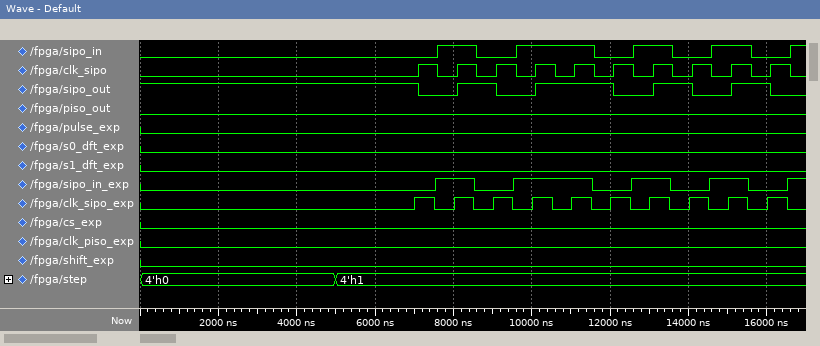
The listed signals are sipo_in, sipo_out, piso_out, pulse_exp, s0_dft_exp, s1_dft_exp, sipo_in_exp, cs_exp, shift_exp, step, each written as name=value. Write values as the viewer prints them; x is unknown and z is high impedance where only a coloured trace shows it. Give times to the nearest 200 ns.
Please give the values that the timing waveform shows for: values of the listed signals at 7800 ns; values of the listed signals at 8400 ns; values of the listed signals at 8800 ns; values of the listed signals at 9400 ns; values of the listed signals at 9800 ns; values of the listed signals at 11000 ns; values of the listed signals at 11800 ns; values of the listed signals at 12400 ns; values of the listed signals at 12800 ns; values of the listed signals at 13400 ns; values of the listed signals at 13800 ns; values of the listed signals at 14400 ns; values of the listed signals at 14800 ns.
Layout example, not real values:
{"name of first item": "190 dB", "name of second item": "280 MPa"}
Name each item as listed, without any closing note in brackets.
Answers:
{"values of the listed signals at 7800 ns": "sipo_in=1, sipo_out=0, piso_out=0, pulse_exp=0, s0_dft_exp=0, s1_dft_exp=0, sipo_in_exp=1, cs_exp=0, shift_exp=0, step=4'h1", "values of the listed signals at 8400 ns": "sipo_in=1, sipo_out=1, piso_out=0, pulse_exp=0, s0_dft_exp=0, s1_dft_exp=0, sipo_in_exp=1, cs_exp=0, shift_exp=0, step=4'h1", "values of the listed signals at 8800 ns": "sipo_in=0, sipo_out=1, piso_out=0, pulse_exp=0, s0_dft_exp=0, s1_dft_exp=0, sipo_in_exp=0, cs_exp=0, shift_exp=0, step=4'h1", "values of the listed signals at 9400 ns": "sipo_in=0, sipo_out=0, piso_out=0, pulse_exp=0, s0_dft_exp=0, s1_dft_exp=0, sipo_in_exp=0, cs_exp=0, shift_exp=0, step=4'h1", "values of the listed signals at 9800 ns": "sipo_in=1, sipo_out=0, piso_out=0, pulse_exp=0, s0_dft_exp=0, s1_dft_exp=0, sipo_in_exp=1, cs_exp=0, shift_exp=0, step=4'h1", "values of the listed signals at 11000 ns": "sipo_in=1, sipo_out=1, piso_out=0, pulse_exp=0, s0_dft_exp=0, s1_dft_exp=0, sipo_in_exp=1, cs_exp=0, shift_exp=0, step=4'h1", "values of the listed signals at 11800 ns": "sipo_in=0, sipo_out=1, piso_out=0, pulse_exp=0, s0_dft_exp=0, s1_dft_exp=0, sipo_in_exp=0, cs_exp=0, shift_exp=0, step=4'h1", "values of the listed signals at 12400 ns": "sipo_in=0, sipo_out=0, piso_out=0, pulse_exp=0, s0_dft_exp=0, s1_dft_exp=0, sipo_in_exp=0, cs_exp=0, shift_exp=0, step=4'h1", "values of the listed signals at 12800 ns": "sipo_in=1, sipo_out=0, piso_out=0, pulse_exp=0, s0_dft_exp=0, s1_dft_exp=0, sipo_in_exp=1, cs_exp=0, shift_exp=0, step=4'h1", "values of the listed signals at 13400 ns": "sipo_in=1, sipo_out=1, piso_out=0, pulse_exp=0, s0_dft_exp=0, s1_dft_exp=0, sipo_in_exp=1, cs_exp=0, shift_exp=0, step=4'h1", "values of the listed signals at 13800 ns": "sipo_in=0, sipo_out=1, piso_out=0, pulse_exp=0, s0_dft_exp=0, s1_dft_exp=0, sipo_in_exp=0, cs_exp=0, shift_exp=0, step=4'h1", "values of the listed signals at 14400 ns": "sipo_in=0, sipo_out=0, piso_out=0, pulse_exp=0, s0_dft_exp=0, s1_dft_exp=0, sipo_in_exp=0, cs_exp=0, shift_exp=0, step=4'h1", "values of the listed signals at 14800 ns": "sipo_in=1, sipo_out=0, piso_out=0, pulse_exp=0, s0_dft_exp=0, s1_dft_exp=0, sipo_in_exp=1, cs_exp=0, shift_exp=0, step=4'h1"}
